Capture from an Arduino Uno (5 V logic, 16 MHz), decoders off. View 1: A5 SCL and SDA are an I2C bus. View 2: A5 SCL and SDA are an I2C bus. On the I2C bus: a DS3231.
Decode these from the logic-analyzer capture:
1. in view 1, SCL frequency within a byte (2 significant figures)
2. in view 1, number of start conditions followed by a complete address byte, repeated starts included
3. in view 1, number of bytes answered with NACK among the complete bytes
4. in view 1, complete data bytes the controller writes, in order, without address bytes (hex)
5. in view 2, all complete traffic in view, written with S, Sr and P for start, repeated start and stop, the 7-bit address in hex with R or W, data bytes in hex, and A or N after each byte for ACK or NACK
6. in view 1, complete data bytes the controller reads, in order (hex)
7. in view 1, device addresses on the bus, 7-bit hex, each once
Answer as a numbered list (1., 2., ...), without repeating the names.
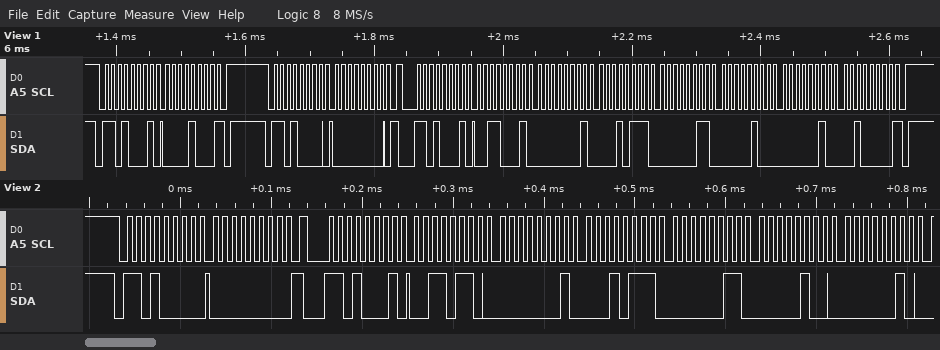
1. 100 kHz
2. 3
3. 2
4. 00
5. S 68W A 00 A Sr 68R A 36 A 01 A 17 A 03 A 04 A 02 A
6. 08 31 01 17 03 04 02 20
7. 0x68
